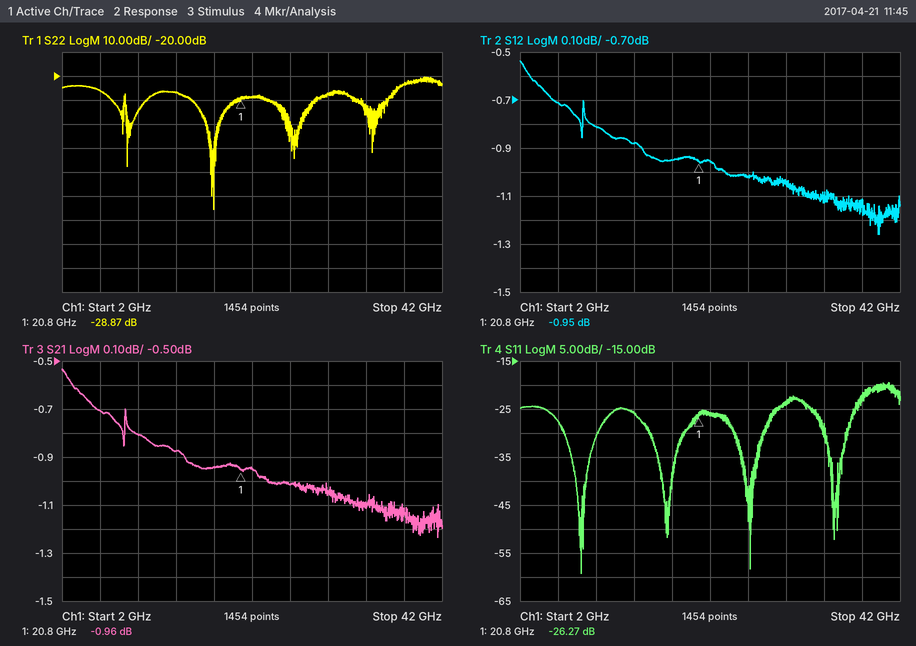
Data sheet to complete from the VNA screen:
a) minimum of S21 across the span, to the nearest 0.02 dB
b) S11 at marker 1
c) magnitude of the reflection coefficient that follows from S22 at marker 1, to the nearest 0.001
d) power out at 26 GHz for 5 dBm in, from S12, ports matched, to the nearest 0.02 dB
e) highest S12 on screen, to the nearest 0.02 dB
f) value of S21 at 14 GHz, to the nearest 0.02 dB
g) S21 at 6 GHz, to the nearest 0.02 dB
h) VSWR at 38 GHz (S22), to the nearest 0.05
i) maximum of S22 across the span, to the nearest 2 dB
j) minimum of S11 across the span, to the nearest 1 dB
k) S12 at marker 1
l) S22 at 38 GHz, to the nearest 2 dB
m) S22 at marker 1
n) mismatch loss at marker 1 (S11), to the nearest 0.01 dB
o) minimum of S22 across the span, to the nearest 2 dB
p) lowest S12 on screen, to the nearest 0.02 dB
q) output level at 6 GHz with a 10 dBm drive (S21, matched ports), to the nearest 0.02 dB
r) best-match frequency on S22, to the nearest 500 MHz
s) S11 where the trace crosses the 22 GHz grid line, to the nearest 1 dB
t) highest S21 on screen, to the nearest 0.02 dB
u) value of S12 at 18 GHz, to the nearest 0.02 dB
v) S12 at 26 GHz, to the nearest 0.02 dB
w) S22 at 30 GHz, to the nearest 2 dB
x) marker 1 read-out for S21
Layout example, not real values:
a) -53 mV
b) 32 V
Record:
a) -1.24 dB
b) -26.27 dB
c) 0.036
d) 3.98 dBm
e) -0.54 dB
f) -0.88 dB
g) -0.70 dB
h) 1.15
i) -20 dB
j) -59 dB
k) -0.95 dB
l) -24 dB
m) -28.87 dB
n) 0.01 dB
o) -76 dB
p) -1.26 dB
q) 9.30 dBm
r) 18.0 GHz
s) -26 dB
t) -0.54 dB
u) -0.96 dB
v) -1.02 dB
w) -28 dB
x) -0.96 dB
